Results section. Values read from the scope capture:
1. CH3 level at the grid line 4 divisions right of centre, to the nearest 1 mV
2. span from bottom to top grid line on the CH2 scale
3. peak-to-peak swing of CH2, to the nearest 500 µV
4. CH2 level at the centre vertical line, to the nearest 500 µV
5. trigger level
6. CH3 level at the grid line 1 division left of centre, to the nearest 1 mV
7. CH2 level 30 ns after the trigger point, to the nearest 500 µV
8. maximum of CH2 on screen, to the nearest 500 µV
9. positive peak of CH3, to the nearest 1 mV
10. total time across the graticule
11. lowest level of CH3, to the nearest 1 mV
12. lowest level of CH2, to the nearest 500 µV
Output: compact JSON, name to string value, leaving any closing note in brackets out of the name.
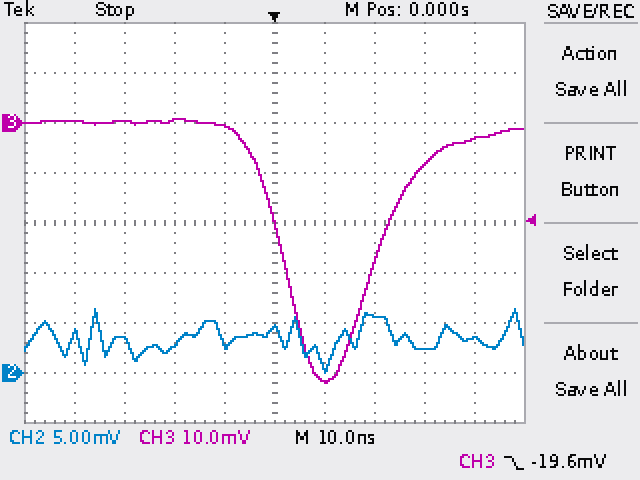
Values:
{"CH3 level at the grid line 4 divisions right of centre, to the nearest 1 mV": "-3 mV", "span from bottom to top grid line on the CH2 scale": "40 mV", "peak-to-peak swing of CH2, to the nearest 500 µV": "6.5 mV", "CH2 level at the centre vertical line, to the nearest 500 µV": "4.5 mV", "trigger level": "-19.6 mV", "CH3 level at the grid line 1 division left of centre, to the nearest 1 mV": "-1 mV", "CH2 level 30 ns after the trigger point, to the nearest 500 µV": "2.5 mV", "maximum of CH2 on screen, to the nearest 500 µV": "6.5 mV", "positive peak of CH3, to the nearest 1 mV": "1 mV", "total time across the graticule": "100 ns", "lowest level of CH3, to the nearest 1 mV": "-52 mV", "lowest level of CH2, to the nearest 500 µV": "0.0 mV"}
